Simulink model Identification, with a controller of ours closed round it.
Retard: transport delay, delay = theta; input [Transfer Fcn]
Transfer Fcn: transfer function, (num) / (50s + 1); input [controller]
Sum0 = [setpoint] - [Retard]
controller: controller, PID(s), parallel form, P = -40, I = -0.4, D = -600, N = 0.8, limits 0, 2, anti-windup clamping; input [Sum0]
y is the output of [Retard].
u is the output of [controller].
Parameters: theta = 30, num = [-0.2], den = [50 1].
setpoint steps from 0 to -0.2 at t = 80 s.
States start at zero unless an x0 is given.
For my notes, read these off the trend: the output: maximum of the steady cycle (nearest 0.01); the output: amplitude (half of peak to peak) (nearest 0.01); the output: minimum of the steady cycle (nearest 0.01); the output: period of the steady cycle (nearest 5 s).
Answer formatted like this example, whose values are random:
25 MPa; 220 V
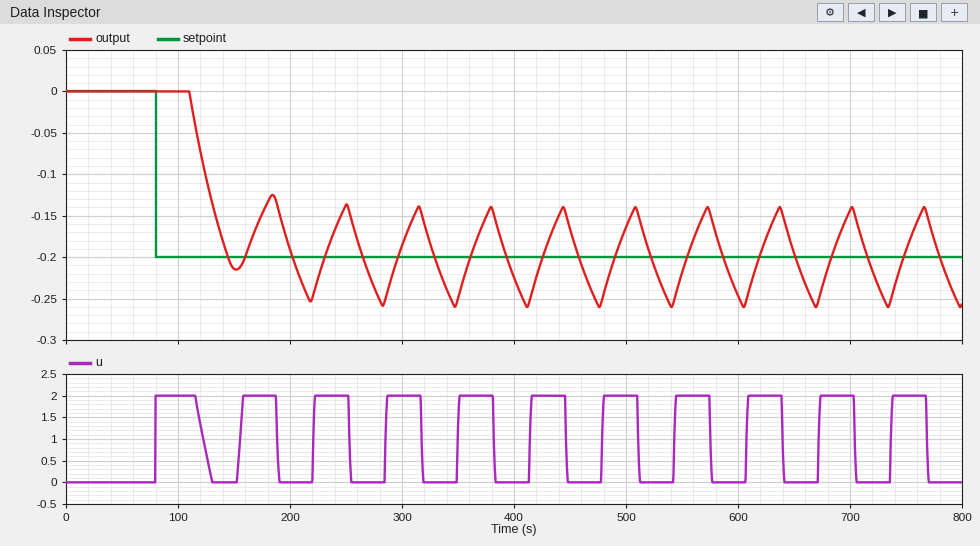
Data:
-0.14; 0.06; -0.26; 65 s
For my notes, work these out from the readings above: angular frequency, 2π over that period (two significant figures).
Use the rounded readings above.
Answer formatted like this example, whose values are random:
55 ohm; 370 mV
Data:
0.097 rad/s
